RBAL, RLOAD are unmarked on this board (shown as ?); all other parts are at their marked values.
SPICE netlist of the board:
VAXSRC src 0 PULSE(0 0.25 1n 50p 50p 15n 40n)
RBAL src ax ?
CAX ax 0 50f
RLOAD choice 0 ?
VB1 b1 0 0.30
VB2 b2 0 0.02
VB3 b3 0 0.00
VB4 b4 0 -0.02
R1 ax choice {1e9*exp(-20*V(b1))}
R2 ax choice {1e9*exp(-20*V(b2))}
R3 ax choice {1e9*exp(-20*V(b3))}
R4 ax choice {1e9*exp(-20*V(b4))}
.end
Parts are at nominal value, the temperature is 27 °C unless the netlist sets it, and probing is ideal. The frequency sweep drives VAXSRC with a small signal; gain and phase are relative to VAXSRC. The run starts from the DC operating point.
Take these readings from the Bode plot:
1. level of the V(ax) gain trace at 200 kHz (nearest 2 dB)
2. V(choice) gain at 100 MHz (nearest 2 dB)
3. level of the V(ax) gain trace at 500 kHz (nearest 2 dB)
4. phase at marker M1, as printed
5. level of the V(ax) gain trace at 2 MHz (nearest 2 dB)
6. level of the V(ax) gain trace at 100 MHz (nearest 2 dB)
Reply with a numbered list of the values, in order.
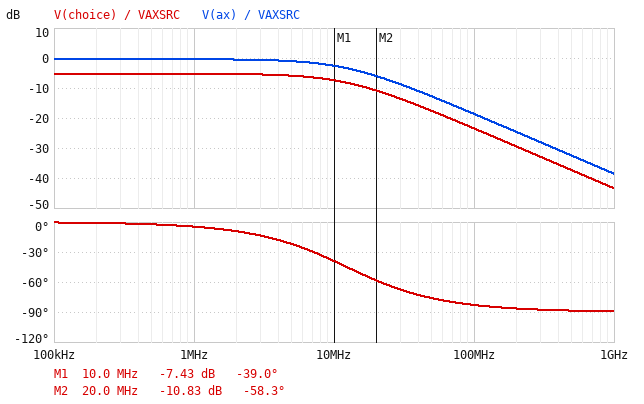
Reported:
1. 0 dB
2. -24 dB
3. 0 dB
4. -39.0 deg
5. 0 dB
6. -18 dB
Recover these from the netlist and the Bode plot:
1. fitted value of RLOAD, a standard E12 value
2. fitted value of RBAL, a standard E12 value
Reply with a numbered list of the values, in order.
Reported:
1. 3.3 MΩ
2. 270 kΩ
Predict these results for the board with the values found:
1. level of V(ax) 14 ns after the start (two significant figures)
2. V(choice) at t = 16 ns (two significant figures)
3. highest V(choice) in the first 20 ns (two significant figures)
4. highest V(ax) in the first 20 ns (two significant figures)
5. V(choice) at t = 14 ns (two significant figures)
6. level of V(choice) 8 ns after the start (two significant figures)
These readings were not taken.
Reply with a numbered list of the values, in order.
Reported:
1. 150 mV
2. 94 mV
3. 94 mV
4. 160 mV
5. 87 mV
6. 57 mV
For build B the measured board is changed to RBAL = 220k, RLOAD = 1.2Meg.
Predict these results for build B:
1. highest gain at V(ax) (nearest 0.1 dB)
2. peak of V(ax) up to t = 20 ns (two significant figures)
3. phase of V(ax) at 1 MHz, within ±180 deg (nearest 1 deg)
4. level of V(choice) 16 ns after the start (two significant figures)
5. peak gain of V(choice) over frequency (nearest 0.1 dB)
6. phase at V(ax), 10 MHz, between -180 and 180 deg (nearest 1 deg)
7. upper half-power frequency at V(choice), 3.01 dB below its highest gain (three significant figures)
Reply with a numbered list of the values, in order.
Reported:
1. -0.5 dB
2. 180 mV
3. -4 deg
4. 59 mV
5. -10.2 dB
6. -33 deg
7. 15.3 MHz
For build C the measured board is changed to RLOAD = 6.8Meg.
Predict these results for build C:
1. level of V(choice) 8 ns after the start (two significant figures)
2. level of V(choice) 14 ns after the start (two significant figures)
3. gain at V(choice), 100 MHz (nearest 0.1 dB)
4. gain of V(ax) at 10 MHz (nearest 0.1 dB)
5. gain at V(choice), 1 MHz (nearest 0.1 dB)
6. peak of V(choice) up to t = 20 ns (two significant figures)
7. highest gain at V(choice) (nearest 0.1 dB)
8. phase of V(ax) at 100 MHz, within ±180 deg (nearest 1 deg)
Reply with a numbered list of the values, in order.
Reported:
1. 74 mV
2. 110 mV
3. -21.3 dB
4. -2.5 dB
5. -3.0 dB
6. 120 mV
7. -2.9 dB
8. -83 deg
